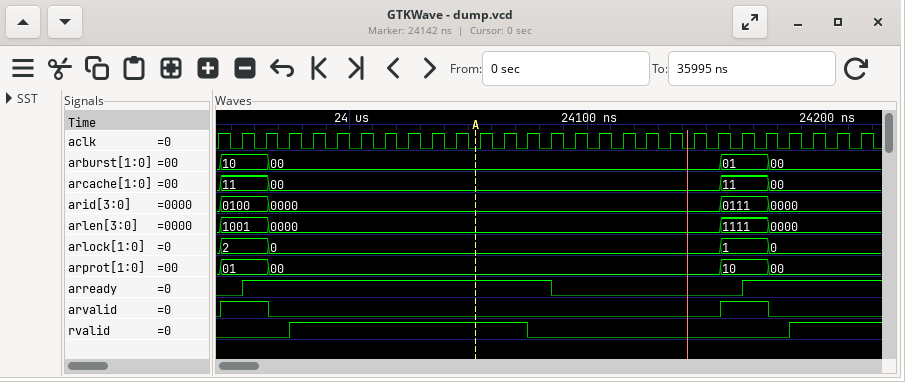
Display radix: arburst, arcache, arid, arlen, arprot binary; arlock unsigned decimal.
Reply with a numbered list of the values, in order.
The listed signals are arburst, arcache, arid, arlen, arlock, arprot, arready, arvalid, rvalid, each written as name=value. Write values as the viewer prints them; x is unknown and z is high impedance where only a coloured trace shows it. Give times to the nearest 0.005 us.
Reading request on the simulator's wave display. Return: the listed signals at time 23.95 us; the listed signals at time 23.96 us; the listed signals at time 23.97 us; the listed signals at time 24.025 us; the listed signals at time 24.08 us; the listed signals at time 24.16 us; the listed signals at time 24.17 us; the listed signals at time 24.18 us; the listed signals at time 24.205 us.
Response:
1. arburst=10, arcache=11, arid=0100, arlen=1001, arlock=2, arprot=01, arready=0, arvalid=1, rvalid=0
2. arburst=10, arcache=11, arid=0100, arlen=1001, arlock=2, arprot=01, arready=1, arvalid=1, rvalid=0
3. arburst=00, arcache=00, arid=0000, arlen=0000, arlock=0, arprot=00, arready=1, arvalid=0, rvalid=0
4. arburst=00, arcache=00, arid=0000, arlen=0000, arlock=0, arprot=00, arready=1, arvalid=0, rvalid=1
5. arburst=00, arcache=00, arid=0000, arlen=0000, arlock=0, arprot=00, arready=1, arvalid=0, rvalid=0
6. arburst=01, arcache=11, arid=0111, arlen=1111, arlock=1, arprot=10, arready=0, arvalid=1, rvalid=0
7. arburst=01, arcache=11, arid=0111, arlen=1111, arlock=1, arprot=10, arready=1, arvalid=1, rvalid=0
8. arburst=00, arcache=00, arid=0000, arlen=0000, arlock=0, arprot=00, arready=1, arvalid=0, rvalid=0
9. arburst=00, arcache=00, arid=0000, arlen=0000, arlock=0, arprot=00, arready=1, arvalid=0, rvalid=1
